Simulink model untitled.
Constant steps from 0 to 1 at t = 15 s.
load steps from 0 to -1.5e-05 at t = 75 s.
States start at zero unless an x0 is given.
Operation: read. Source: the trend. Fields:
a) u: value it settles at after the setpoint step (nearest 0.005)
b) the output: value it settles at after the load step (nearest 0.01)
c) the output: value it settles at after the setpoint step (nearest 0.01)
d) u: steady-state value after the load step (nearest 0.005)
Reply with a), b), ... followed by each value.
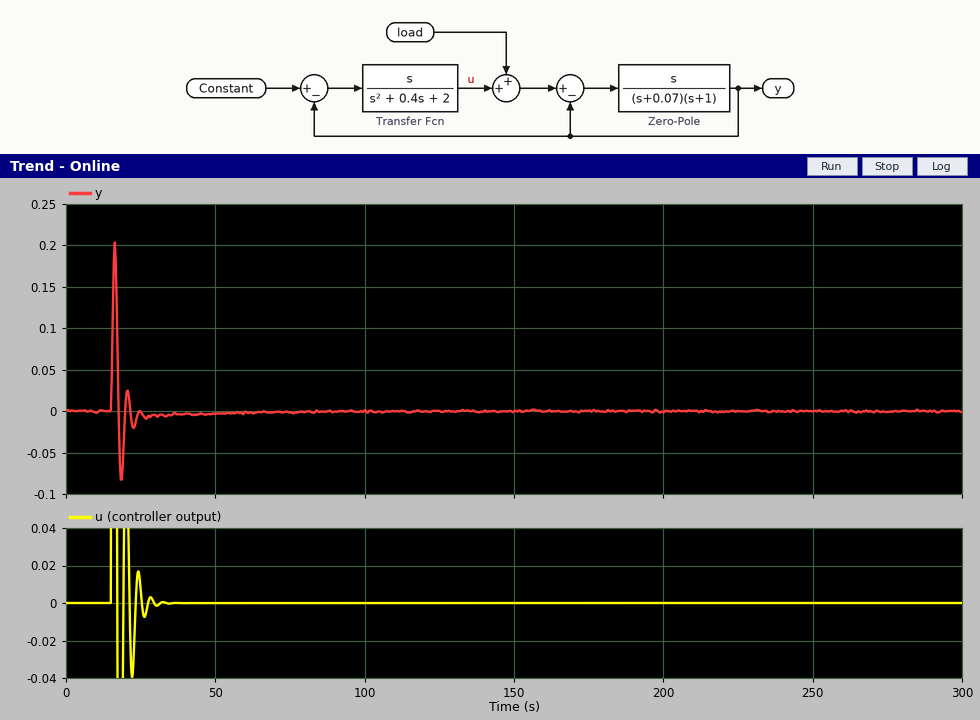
a) 0.000
b) 0.00
c) 0.00
d) 0.000
